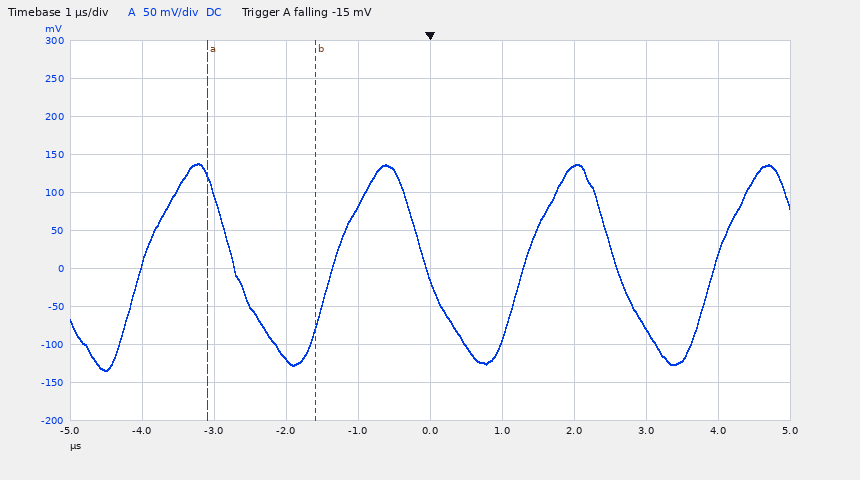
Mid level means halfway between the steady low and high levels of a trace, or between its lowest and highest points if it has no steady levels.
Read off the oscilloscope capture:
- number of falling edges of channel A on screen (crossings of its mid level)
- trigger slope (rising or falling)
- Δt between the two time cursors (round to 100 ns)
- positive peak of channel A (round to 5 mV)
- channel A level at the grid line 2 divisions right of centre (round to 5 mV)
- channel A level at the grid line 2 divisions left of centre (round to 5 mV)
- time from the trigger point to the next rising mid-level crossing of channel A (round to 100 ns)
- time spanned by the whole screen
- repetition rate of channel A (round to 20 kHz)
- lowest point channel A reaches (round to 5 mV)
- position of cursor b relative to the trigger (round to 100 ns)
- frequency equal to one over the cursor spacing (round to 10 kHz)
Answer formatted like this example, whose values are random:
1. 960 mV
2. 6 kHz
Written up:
1. 3
2. falling
3. 1.5 µs
4. 140 mV
5. 135 mV
6. -120 mV
7. 1.3 µs
8. 10 µs
9. 380 kHz
10. -135 mV
11. -1.6 µs
12. 670 kHz
